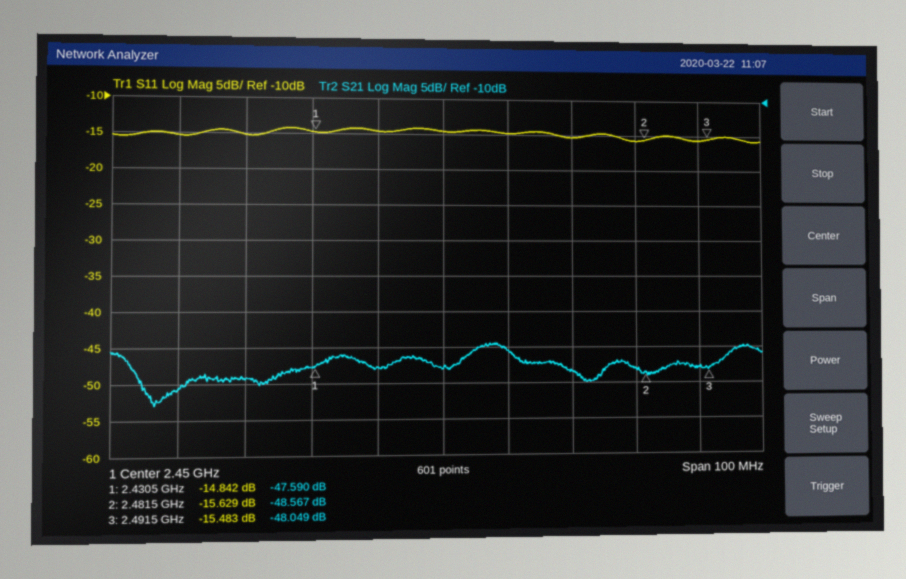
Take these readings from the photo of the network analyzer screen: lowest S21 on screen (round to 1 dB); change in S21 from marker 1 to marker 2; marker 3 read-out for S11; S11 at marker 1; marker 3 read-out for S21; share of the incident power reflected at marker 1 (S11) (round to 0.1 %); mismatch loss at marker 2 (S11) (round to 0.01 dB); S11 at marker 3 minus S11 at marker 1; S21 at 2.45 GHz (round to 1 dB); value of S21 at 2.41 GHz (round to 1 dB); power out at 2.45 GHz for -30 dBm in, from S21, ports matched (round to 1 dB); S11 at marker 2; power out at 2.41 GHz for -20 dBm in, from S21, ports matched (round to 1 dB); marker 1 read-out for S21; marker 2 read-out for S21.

-53 dB
-0.977 dB
-15.483 dB
-14.842 dB
-48.049 dB
3.3 %
0.12 dB
-0.641 dB
-48 dB
-51 dB
-78 dBm
-15.629 dB
-71 dBm
-47.590 dB
-48.567 dB
